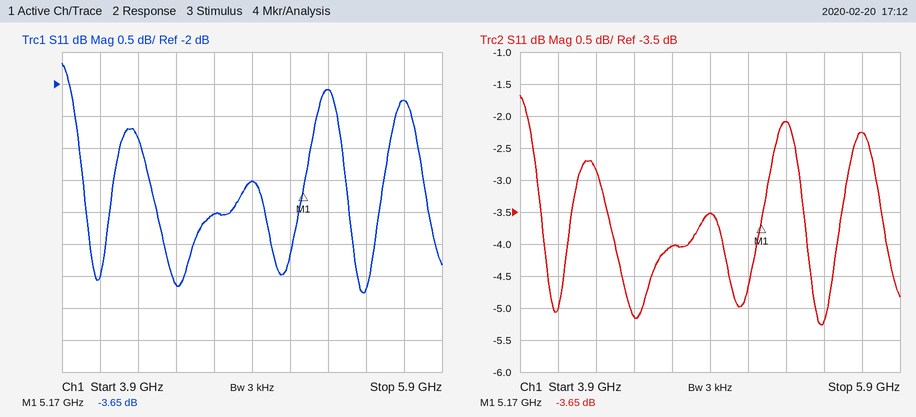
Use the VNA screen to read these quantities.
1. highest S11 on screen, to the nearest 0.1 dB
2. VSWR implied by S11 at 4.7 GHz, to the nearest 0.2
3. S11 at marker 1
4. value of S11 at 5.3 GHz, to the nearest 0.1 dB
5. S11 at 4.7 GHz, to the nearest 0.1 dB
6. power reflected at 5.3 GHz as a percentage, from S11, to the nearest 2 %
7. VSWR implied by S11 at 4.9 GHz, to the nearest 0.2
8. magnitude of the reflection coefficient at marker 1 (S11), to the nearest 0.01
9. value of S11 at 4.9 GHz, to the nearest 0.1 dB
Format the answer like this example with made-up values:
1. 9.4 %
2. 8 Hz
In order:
1. -1.7 dB
2. 4.4
3. -3.65 dB
4. -2.1 dB
5. -4.0 dB
6. 62 %
7. 5.0
8. 0.66
9. -3.5 dB
